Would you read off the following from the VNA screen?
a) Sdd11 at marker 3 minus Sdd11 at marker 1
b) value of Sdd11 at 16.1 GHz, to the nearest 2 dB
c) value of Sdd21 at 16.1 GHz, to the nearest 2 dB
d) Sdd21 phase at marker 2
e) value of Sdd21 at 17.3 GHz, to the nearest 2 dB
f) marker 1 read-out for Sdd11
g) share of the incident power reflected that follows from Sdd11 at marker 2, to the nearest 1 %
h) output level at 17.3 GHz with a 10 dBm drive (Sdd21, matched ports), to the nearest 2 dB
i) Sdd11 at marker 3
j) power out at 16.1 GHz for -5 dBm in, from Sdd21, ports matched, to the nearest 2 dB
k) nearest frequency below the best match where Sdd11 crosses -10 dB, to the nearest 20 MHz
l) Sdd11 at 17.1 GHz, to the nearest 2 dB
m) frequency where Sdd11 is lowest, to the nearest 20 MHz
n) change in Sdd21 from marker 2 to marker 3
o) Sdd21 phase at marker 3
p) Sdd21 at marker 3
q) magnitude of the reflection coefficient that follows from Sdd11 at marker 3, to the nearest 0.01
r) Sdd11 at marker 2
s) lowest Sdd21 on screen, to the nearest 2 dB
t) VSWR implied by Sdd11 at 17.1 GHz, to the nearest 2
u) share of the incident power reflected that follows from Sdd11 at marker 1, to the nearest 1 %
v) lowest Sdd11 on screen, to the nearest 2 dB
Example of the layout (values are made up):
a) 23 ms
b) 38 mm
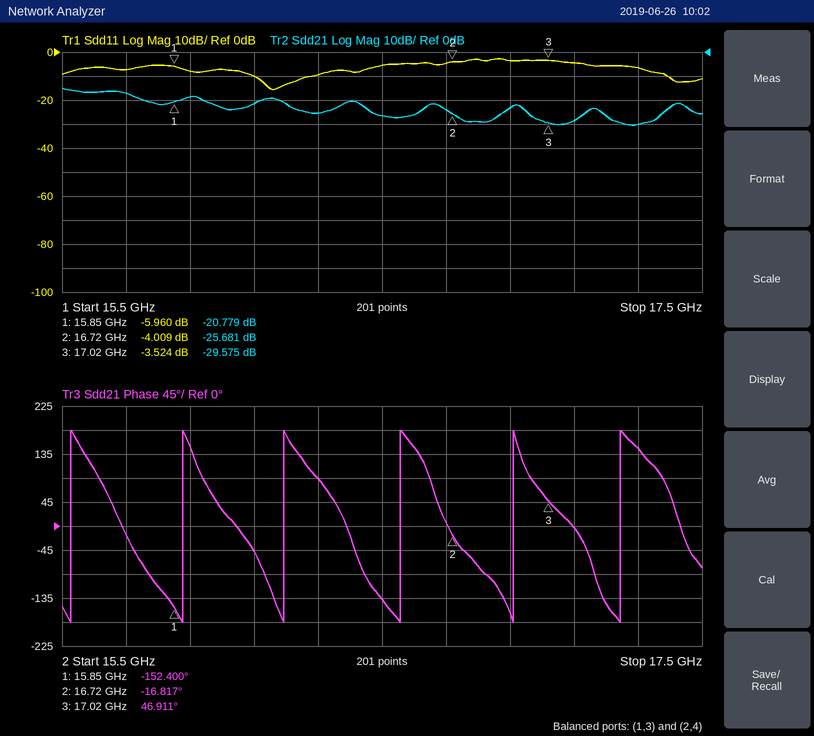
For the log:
a) 2.436 dB
b) -10 dB
c) -22 dB
d) -16.817°
e) -30 dB
f) -5.960 dB
g) 40 %
h) -20 dBm
i) -3.524 dB
j) -26 dBm
k) 16.10 GHz
l) -4 dB
m) 16.16 GHz
n) -3.894 dB
o) 46.911°
p) -29.575 dB
q) 0.67
r) -4.009 dB
s) -30 dB
t) 4
u) 25 %
v) -16 dB
